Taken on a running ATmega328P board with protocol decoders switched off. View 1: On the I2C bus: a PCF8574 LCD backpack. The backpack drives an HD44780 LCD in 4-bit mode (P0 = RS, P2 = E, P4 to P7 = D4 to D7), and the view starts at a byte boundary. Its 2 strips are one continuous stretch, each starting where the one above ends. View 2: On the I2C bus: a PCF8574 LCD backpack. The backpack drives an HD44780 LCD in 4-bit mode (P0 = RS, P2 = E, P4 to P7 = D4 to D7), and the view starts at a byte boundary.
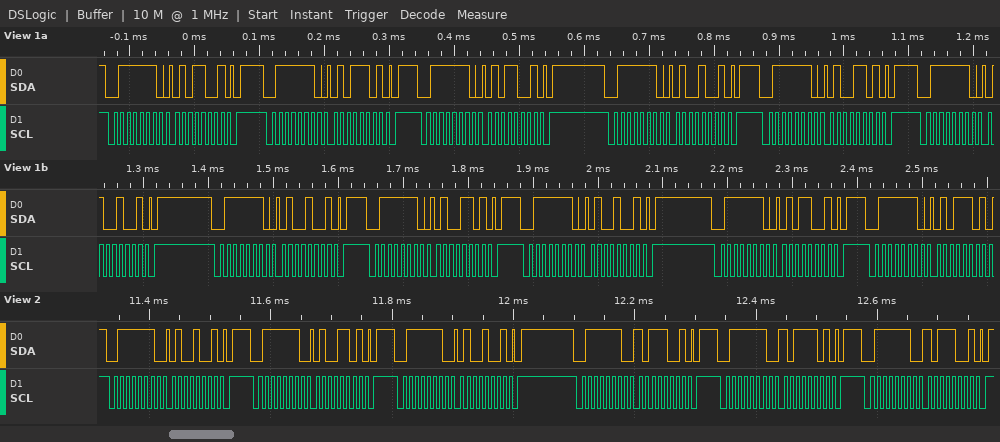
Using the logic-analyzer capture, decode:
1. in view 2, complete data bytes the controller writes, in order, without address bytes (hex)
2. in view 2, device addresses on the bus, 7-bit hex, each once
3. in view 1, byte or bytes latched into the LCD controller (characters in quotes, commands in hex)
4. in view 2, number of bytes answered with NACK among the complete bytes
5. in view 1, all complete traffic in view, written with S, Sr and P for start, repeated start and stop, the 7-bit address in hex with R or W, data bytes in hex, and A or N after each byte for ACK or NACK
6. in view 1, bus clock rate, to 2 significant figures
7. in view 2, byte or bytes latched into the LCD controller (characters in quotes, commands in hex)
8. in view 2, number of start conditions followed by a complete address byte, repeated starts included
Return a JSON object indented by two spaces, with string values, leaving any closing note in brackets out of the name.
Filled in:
{
  "in view 2, complete data bytes the controller writes, in order, without address bytes": "49 4D 49 B9 BD B9",
  "in view 2, device addresses on the bus, 7-bit hex, each once": "0x3F",
  "in view 1, byte or bytes latched into the LCD controller": "'T'",
  "in view 2, number of bytes answered with NACK among the complete bytes": "0",
  "in view 1, all complete traffic in view, written with S, Sr and P for start, repeated start and stop, the 7-bit address in hex with R or W, data bytes in hex, and A or N after each byte for ACK or NACK": "S 3FW A 59 A P S 3FW A 5D A P S 3FW A 59 A P S 3FW A 49 A P S 3FW A 4D A P S 3FW A 49 A P S 3FW A 49 A P S 3FW A 4D A P S 3FW A 49 A P S 3FW A 59 A P S 3FW A 5D A",
  "in view 1, bus clock rate, to 2 significant figures": "100 kHz",
  "in view 2, byte or bytes latched into the LCD controller": "'K'",
  "in view 2, number of start conditions followed by a complete address byte, repeated starts included": "6"
}
